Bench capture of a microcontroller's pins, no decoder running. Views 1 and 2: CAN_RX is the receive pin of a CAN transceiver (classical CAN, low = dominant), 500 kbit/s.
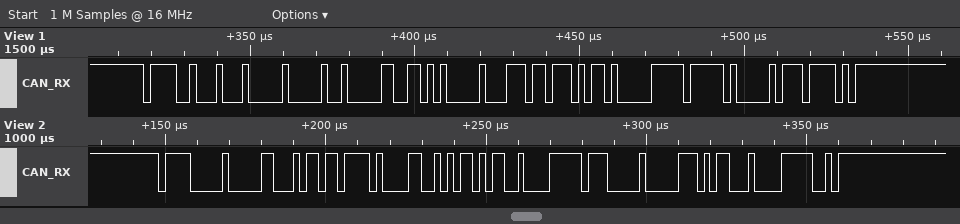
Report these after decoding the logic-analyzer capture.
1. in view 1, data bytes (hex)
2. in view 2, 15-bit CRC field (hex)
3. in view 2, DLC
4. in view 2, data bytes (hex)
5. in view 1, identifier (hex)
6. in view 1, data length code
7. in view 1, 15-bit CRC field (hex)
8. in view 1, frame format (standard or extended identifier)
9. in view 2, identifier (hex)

00 41 35 00 ED D6 83 FF
0x443E
8
B6 F4 32 B5 90 FF 00 35
0x791
8
0x01DE
standard
0x780
